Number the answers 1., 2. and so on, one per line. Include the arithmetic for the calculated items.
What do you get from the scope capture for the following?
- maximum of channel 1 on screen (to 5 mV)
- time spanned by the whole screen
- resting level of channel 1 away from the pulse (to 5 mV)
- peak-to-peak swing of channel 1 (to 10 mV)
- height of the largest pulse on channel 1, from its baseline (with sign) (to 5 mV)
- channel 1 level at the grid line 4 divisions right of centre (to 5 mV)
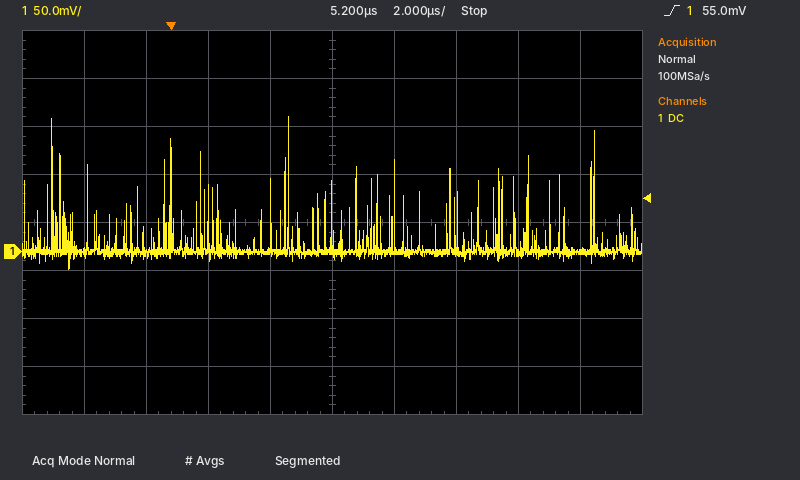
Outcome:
1. 140 mV
2. 20 µs
3. 0 mV
4. 160 mV
5. 140 mV − (0 mV) = +140 mV
6. 0 mV
